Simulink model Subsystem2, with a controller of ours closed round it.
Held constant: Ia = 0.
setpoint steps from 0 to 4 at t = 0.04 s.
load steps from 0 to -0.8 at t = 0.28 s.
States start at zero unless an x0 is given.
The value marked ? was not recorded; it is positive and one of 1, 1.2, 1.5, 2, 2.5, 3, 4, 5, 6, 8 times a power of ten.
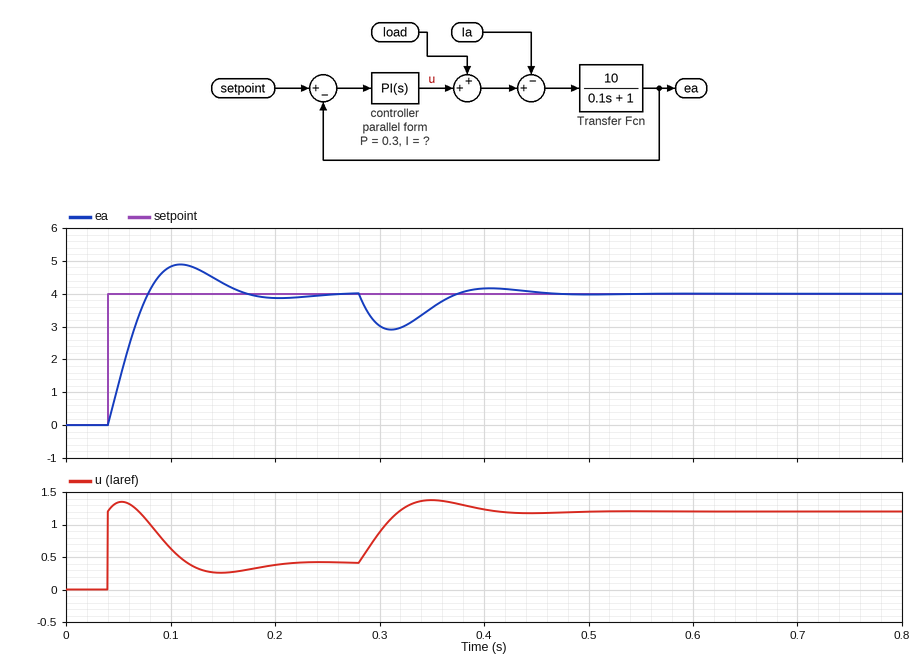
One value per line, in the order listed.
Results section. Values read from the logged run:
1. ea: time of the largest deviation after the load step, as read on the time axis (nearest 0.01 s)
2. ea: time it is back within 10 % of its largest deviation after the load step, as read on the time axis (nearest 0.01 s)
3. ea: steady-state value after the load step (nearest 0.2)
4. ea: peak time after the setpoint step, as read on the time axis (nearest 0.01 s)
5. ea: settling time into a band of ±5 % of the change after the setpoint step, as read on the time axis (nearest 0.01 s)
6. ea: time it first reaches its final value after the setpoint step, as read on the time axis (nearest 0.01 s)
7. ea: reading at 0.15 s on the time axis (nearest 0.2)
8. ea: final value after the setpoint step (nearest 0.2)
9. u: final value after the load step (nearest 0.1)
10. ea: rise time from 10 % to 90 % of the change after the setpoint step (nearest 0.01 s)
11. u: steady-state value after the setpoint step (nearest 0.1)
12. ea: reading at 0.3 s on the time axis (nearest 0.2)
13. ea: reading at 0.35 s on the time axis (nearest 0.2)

0.31 s
0.43 s
4.0
0.11 s
0.16 s
0.08 s
4.4
4.0
1.2
0.03 s
0.4
3.0
3.6
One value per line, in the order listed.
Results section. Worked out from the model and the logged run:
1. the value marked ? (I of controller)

15
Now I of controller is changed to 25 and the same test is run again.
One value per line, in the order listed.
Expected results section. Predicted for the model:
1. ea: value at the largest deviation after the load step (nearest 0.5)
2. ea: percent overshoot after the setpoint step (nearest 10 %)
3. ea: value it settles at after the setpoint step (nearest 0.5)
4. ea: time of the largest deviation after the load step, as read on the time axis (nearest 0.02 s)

3.0
30 %
4.0
0.30 s
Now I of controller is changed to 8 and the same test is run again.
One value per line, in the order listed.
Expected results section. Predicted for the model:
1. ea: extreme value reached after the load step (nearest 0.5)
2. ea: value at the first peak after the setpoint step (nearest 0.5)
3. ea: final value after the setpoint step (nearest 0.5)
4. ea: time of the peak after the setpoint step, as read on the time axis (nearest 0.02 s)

2.5
4.5
4.0
0.14 s
